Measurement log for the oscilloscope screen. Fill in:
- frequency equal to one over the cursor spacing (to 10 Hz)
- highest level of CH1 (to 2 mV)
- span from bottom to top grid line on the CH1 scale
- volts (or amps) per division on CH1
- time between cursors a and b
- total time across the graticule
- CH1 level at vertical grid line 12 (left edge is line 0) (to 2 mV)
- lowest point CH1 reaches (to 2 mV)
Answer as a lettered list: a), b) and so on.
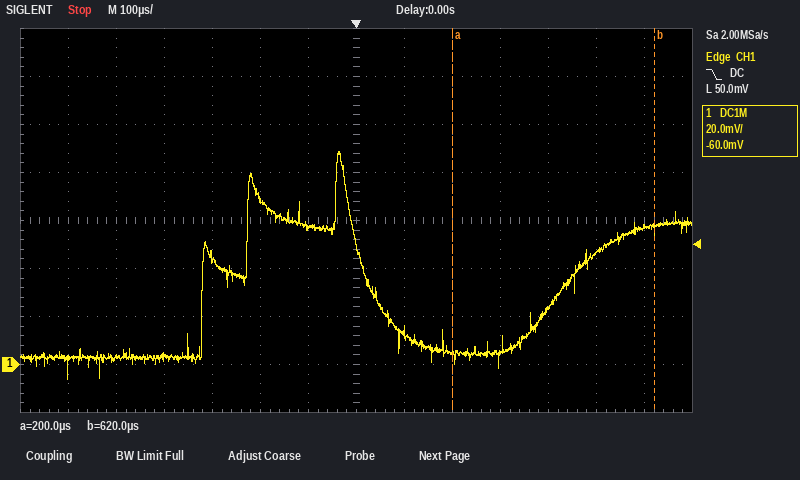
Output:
a) 2.38 kHz
b) 88 mV
c) 160 mV
d) 20 mV
e) 420 µs
f) 1.4 ms
g) 46 mV
h) -6 mV
